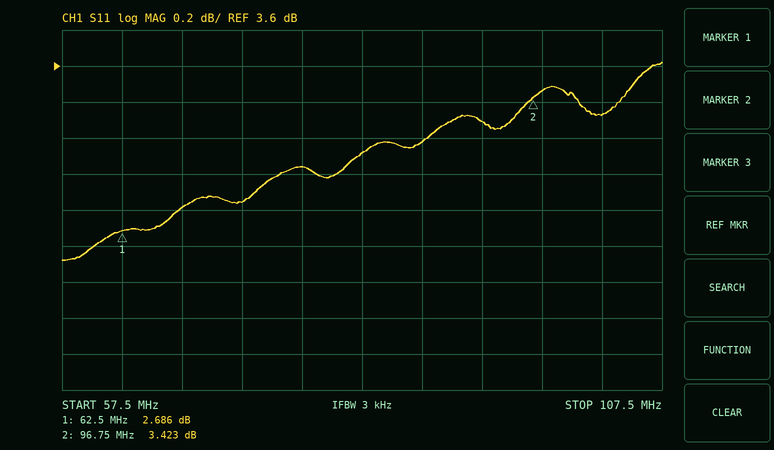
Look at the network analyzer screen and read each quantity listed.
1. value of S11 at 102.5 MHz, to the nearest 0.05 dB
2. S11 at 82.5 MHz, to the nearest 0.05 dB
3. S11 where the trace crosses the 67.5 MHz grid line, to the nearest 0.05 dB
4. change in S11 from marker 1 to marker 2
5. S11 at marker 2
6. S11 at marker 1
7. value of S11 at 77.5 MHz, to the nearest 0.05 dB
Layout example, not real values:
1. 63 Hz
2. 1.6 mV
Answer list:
1. 3.35 dB
2. 3.10 dB
3. 2.80 dB
4. 0.737 dB
5. 3.423 dB
6. 2.686 dB
7. 3.05 dB
